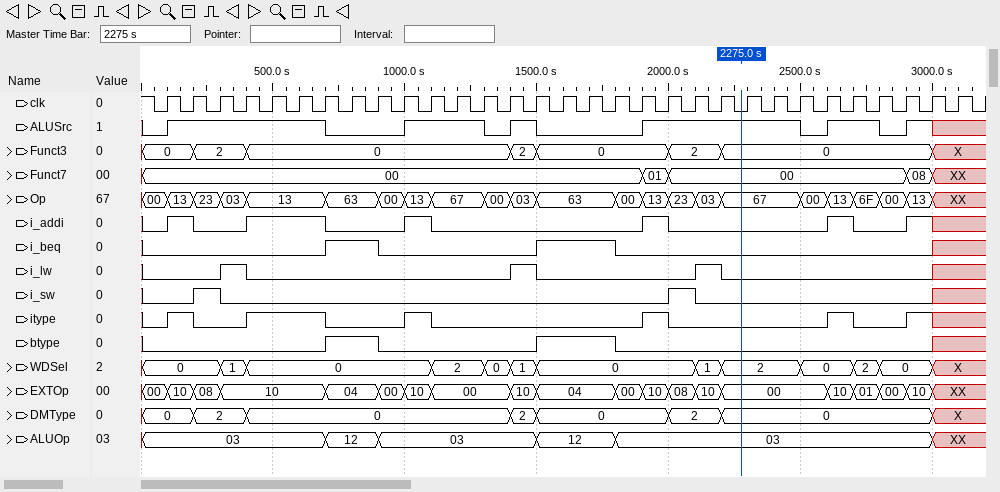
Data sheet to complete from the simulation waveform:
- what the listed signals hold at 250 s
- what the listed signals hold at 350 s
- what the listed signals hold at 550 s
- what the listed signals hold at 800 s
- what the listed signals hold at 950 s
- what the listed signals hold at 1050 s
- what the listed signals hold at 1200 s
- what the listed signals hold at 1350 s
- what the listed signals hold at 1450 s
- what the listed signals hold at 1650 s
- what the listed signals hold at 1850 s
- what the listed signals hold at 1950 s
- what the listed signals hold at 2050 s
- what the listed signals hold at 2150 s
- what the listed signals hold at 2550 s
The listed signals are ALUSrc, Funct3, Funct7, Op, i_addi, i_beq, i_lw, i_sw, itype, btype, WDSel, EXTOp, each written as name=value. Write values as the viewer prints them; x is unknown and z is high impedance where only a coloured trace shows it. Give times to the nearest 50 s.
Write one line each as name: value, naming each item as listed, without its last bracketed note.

what the listed signals hold at 250 s: ALUSrc=1, Funct3=2, Funct7=00, Op=23, i_addi=0, i_beq=0, i_lw=0, i_sw=1, itype=0, btype=0, WDSel=0, EXTOp=08
what the listed signals hold at 350 s: ALUSrc=1, Funct3=2, Funct7=00, Op=03, i_addi=0, i_beq=0, i_lw=1, i_sw=0, itype=0, btype=0, WDSel=1, EXTOp=10
what the listed signals hold at 550 s: ALUSrc=1, Funct3=0, Funct7=00, Op=13, i_addi=1, i_beq=0, i_lw=0, i_sw=0, itype=1, btype=0, WDSel=0, EXTOp=10
what the listed signals hold at 800 s: ALUSrc=0, Funct3=0, Funct7=00, Op=63, i_addi=0, i_beq=1, i_lw=0, i_sw=0, itype=0, btype=1, WDSel=0, EXTOp=04
what the listed signals hold at 950 s: ALUSrc=0, Funct3=0, Funct7=00, Op=00, i_addi=0, i_beq=0, i_lw=0, i_sw=0, itype=0, btype=0, WDSel=0, EXTOp=00
what the listed signals hold at 1050 s: ALUSrc=1, Funct3=0, Funct7=00, Op=13, i_addi=1, i_beq=0, i_lw=0, i_sw=0, itype=1, btype=0, WDSel=0, EXTOp=10
what the listed signals hold at 1200 s: ALUSrc=1, Funct3=0, Funct7=00, Op=67, i_addi=0, i_beq=0, i_lw=0, i_sw=0, itype=0, btype=0, WDSel=2, EXTOp=00
what the listed signals hold at 1350 s: ALUSrc=0, Funct3=0, Funct7=00, Op=00, i_addi=0, i_beq=0, i_lw=0, i_sw=0, itype=0, btype=0, WDSel=0, EXTOp=00
what the listed signals hold at 1450 s: ALUSrc=1, Funct3=2, Funct7=00, Op=03, i_addi=0, i_beq=0, i_lw=1, i_sw=0, itype=0, btype=0, WDSel=1, EXTOp=10
what the listed signals hold at 1650 s: ALUSrc=0, Funct3=0, Funct7=00, Op=63, i_addi=0, i_beq=1, i_lw=0, i_sw=0, itype=0, btype=1, WDSel=0, EXTOp=04
what the listed signals hold at 1850 s: ALUSrc=0, Funct3=0, Funct7=00, Op=00, i_addi=0, i_beq=0, i_lw=0, i_sw=0, itype=0, btype=0, WDSel=0, EXTOp=00
what the listed signals hold at 1950 s: ALUSrc=1, Funct3=0, Funct7=01, Op=13, i_addi=1, i_beq=0, i_lw=0, i_sw=0, itype=1, btype=0, WDSel=0, EXTOp=10
what the listed signals hold at 2050 s: ALUSrc=1, Funct3=2, Funct7=00, Op=23, i_addi=0, i_beq=0, i_lw=0, i_sw=1, itype=0, btype=0, WDSel=0, EXTOp=08
what the listed signals hold at 2150 s: ALUSrc=1, Funct3=2, Funct7=00, Op=03, i_addi=0, i_beq=0, i_lw=1, i_sw=0, itype=0, btype=0, WDSel=1, EXTOp=10
what the listed signals hold at 2550 s: ALUSrc=0, Funct3=0, Funct7=00, Op=00, i_addi=0, i_beq=0, i_lw=0, i_sw=0, itype=0, btype=0, WDSel=0, EXTOp=00
